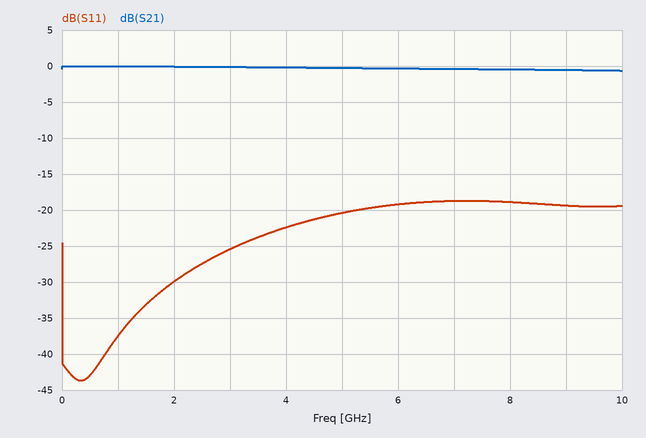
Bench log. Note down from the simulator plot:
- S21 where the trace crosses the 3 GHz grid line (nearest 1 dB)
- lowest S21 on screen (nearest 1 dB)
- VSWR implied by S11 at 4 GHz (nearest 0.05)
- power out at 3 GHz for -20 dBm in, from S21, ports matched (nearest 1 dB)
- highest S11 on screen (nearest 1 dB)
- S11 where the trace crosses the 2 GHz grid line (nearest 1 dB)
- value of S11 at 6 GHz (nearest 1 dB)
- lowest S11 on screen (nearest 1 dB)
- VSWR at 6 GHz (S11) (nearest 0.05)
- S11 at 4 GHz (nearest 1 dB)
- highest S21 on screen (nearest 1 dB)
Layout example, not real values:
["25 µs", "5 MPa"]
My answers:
["0 dB", "-1 dB", "1.15", "-20 dBm", "-19 dB", "-30 dB", "-19 dB", "-44 dB", "1.25", "-22 dB", "0 dB"]
